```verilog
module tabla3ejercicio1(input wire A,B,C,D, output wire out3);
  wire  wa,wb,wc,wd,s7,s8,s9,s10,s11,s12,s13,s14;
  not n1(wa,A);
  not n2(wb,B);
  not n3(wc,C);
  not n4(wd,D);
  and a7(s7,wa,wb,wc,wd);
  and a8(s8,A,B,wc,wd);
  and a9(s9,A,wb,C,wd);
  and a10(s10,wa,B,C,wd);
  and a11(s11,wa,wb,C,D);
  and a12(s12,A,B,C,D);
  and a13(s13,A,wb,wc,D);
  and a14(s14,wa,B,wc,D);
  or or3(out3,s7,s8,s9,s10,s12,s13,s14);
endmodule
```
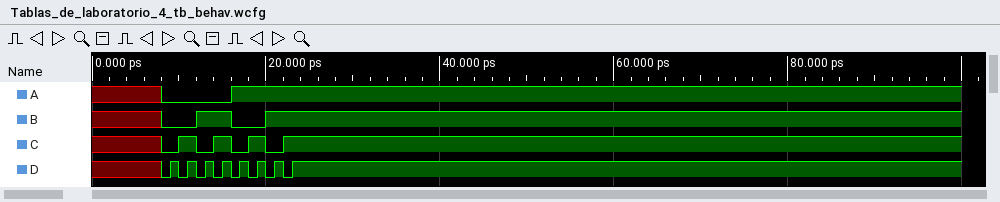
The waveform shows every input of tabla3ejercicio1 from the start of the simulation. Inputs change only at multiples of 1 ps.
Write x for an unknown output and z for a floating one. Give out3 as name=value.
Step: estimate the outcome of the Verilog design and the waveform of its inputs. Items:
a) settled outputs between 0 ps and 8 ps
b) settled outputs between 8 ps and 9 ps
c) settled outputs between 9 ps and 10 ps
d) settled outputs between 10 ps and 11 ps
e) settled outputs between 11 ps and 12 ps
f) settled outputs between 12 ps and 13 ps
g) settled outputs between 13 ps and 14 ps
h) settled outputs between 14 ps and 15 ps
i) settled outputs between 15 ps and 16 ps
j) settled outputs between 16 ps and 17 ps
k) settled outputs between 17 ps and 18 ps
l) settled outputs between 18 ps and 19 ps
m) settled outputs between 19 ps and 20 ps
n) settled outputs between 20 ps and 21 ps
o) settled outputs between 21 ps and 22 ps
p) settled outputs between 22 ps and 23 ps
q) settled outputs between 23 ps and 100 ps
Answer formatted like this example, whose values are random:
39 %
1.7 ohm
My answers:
out3=x
out3=1
out3=0
out3=0
out3=0
out3=0
out3=1
out3=1
out3=0
out3=0
out3=1
out3=1
out3=0
out3=1
out3=0
out3=0
out3=1
